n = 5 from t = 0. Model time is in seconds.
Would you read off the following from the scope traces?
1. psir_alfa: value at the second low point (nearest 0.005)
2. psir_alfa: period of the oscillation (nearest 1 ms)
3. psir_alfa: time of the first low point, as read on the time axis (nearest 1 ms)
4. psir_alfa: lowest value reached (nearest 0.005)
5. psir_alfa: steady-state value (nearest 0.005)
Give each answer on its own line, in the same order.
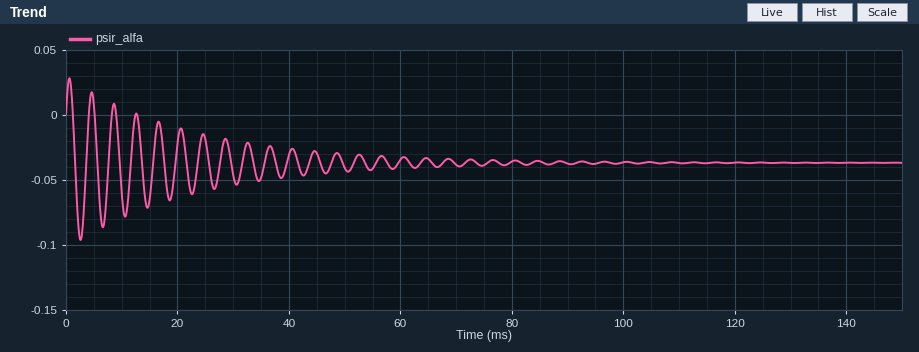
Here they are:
-0.085
4 ms
3 ms
-0.095
-0.035
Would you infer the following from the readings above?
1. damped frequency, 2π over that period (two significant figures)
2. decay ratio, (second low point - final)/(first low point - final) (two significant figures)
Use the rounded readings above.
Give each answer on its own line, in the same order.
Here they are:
1.6 rad/ms
0.83
